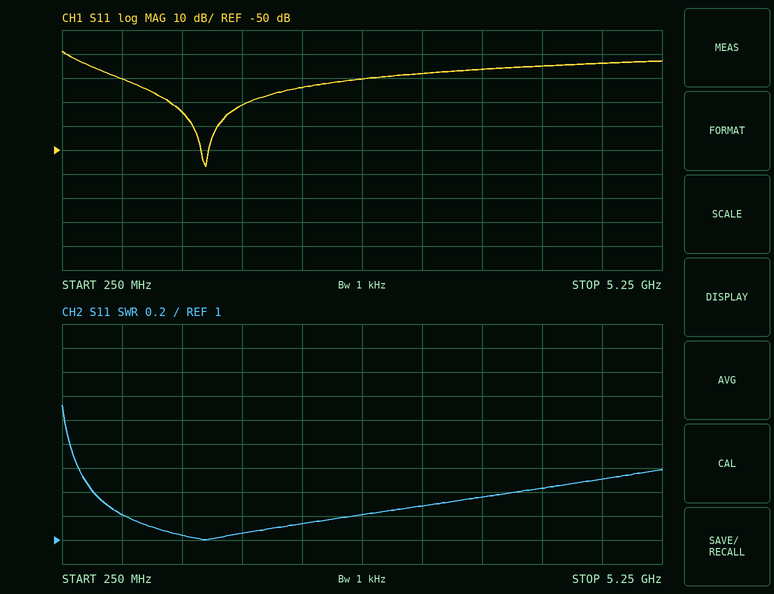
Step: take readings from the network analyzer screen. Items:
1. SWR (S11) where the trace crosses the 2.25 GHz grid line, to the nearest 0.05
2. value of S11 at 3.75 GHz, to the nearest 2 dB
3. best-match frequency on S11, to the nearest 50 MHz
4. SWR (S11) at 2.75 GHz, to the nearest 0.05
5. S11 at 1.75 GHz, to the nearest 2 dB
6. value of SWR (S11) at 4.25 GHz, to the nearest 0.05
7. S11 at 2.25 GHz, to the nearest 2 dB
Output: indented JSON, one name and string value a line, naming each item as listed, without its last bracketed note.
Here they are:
{
  "SWR (S11) where the trace crosses the 2.25 GHz grid line, to the nearest 0.05": "1.15",
  "value of S11 at 3.75 GHz, to the nearest 2 dB": "-16 dB",
  "best-match frequency on S11, to the nearest 50 MHz": "1.45 GHz",
  "SWR (S11) at 2.75 GHz, to the nearest 0.05": "1.20",
  "S11 at 1.75 GHz, to the nearest 2 dB": "-32 dB",
  "value of SWR (S11) at 4.25 GHz, to the nearest 0.05": "1.45",
  "S11 at 2.25 GHz, to the nearest 2 dB": "-24 dB"
}
